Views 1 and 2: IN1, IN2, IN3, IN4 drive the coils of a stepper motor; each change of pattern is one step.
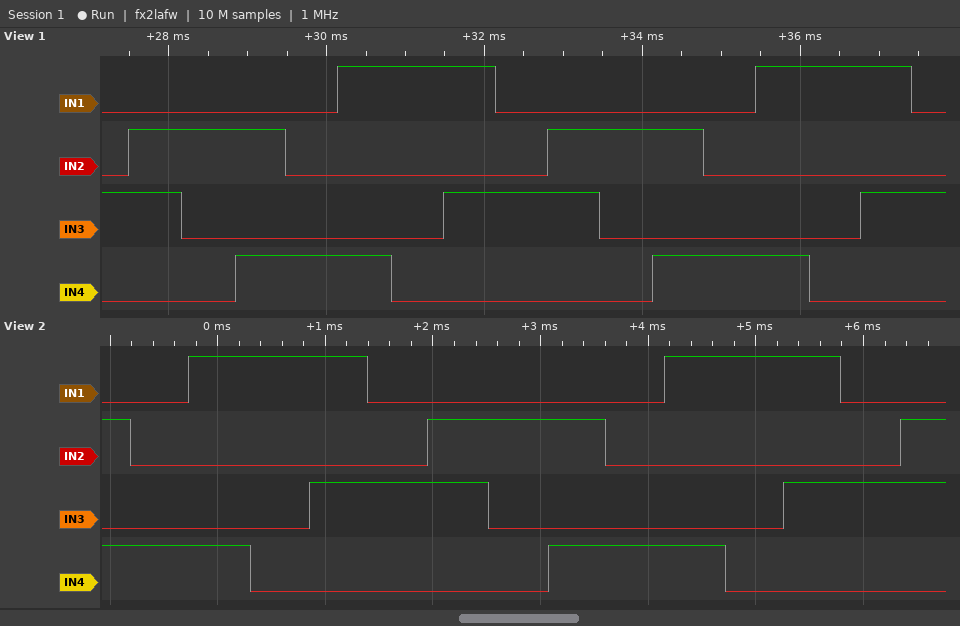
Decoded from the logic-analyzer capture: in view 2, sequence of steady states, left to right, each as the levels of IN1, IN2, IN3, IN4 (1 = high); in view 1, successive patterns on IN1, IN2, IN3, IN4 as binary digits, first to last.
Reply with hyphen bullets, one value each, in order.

- 0101 0001 1001 1000 1010 0010 0110 0100 0101 0001 1001 1000 1010 0010 0110
- 0010 0110 0100 0101 0001 1001 1000 1010 0010 0110 0100 0101 0001 1001 1000 1010 0010
